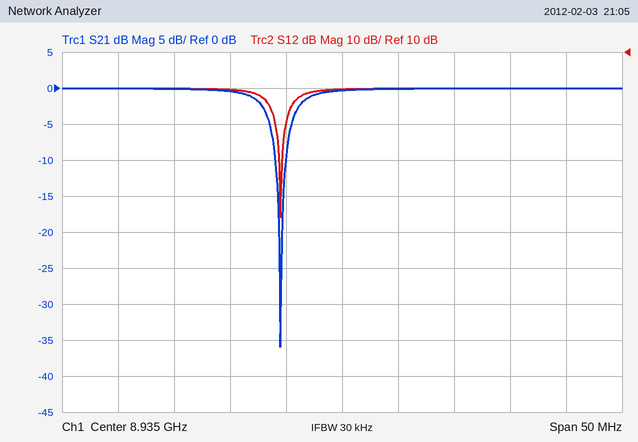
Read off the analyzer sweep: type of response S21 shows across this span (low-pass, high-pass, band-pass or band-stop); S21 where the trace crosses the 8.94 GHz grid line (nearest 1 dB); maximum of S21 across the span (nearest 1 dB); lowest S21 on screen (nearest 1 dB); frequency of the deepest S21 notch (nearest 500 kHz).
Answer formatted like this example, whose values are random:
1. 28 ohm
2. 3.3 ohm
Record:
1. band-stop
2. 0 dB
3. 0 dB
4. -36 dB
5. 8.9295 GHz
